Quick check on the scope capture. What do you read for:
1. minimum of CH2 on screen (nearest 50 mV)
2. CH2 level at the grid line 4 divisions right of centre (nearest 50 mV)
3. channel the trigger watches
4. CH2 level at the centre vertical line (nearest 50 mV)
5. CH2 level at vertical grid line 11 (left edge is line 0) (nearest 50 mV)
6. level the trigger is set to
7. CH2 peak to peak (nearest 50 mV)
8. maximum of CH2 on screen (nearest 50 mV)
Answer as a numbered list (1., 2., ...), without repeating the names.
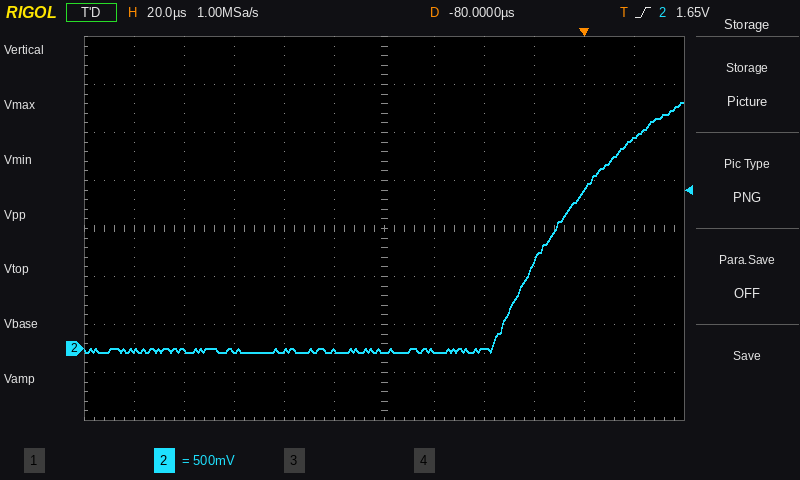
1. -50 mV
2. 1.65 V
3. CH2
4. -50 mV
5. 2.20 V
6. 1.65 V
7. 2.60 V
8. 2.55 V
